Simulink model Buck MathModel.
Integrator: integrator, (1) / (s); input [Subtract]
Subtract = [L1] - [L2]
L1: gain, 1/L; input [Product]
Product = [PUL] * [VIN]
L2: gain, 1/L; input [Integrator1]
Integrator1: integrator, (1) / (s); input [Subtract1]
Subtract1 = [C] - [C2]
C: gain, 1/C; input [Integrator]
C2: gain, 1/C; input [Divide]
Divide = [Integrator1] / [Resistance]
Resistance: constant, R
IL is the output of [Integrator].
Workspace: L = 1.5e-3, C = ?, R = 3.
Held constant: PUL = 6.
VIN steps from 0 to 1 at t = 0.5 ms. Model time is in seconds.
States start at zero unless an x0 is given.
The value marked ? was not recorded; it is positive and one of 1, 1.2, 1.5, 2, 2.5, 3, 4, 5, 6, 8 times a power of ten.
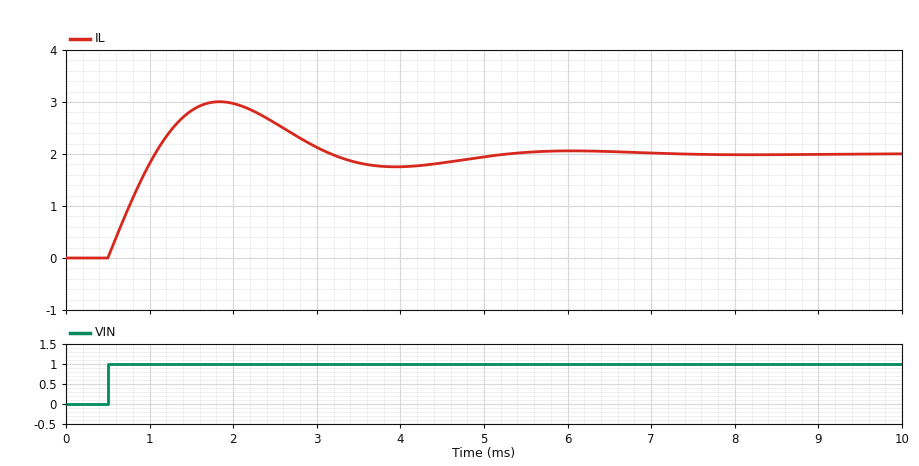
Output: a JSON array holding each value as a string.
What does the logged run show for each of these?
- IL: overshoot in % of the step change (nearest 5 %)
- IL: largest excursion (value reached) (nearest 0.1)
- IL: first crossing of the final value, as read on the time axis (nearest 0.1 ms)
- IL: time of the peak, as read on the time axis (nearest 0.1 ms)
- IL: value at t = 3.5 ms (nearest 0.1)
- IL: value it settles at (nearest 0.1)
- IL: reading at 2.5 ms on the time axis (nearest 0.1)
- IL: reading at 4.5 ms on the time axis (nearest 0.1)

["50 %", "3.0", "1.1 ms", "1.8 ms", "1.8", "2.0", "2.6", "1.8"]
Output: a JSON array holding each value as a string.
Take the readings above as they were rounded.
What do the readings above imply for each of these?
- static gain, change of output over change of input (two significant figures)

["2.0"]
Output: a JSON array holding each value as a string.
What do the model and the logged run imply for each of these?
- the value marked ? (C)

["0.00025"]
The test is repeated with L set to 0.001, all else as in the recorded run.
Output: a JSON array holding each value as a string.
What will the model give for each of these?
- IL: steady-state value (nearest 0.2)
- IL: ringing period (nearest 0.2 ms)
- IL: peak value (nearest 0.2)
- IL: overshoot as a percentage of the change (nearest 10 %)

["2.0", "3.4 ms", "3.6", "80 %"]
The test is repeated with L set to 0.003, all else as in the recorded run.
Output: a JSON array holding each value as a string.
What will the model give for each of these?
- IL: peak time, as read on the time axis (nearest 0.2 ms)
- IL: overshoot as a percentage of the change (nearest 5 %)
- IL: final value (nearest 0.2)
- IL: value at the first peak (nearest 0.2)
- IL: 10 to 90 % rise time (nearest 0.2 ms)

["2.8 ms", "20 %", "2.0", "2.4", "1.0 ms"]
